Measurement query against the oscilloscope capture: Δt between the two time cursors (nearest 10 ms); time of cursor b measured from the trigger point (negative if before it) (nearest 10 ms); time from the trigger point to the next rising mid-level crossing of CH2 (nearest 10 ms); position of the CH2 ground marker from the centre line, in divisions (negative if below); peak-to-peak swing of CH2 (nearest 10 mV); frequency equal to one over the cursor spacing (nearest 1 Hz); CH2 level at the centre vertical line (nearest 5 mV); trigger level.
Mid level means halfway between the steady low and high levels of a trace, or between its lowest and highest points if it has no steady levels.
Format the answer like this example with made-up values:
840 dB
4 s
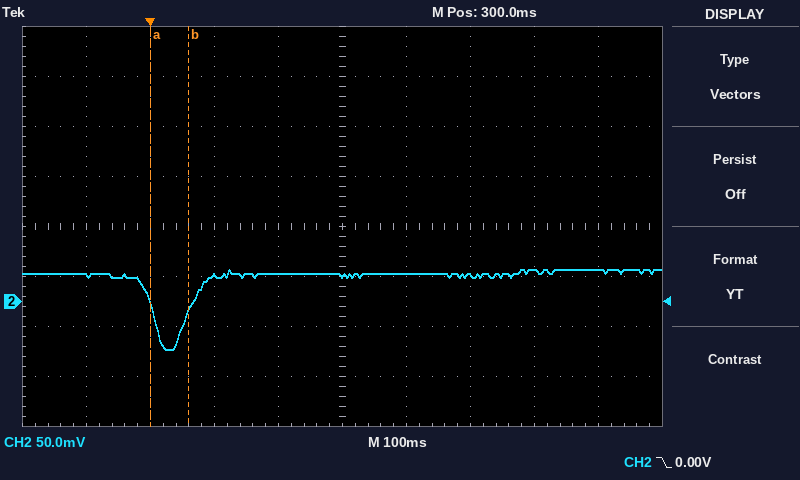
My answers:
60 ms
+60 ms
60 ms
-1.5 div
80 mV
17 Hz
25 mV
0.00 V
